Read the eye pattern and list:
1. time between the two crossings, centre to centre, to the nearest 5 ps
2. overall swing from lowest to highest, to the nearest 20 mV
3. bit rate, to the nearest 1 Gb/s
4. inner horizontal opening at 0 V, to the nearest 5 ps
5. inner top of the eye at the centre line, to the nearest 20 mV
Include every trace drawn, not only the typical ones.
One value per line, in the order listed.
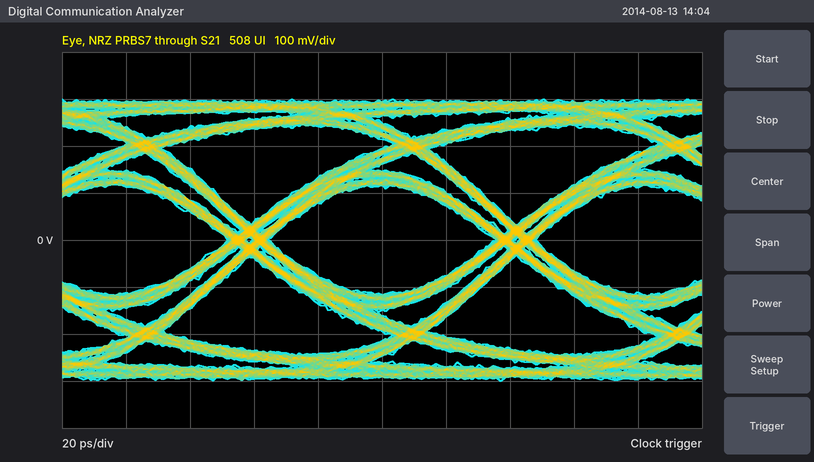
85 ps
600 mV
12 Gb/s
70 ps
120 mV
